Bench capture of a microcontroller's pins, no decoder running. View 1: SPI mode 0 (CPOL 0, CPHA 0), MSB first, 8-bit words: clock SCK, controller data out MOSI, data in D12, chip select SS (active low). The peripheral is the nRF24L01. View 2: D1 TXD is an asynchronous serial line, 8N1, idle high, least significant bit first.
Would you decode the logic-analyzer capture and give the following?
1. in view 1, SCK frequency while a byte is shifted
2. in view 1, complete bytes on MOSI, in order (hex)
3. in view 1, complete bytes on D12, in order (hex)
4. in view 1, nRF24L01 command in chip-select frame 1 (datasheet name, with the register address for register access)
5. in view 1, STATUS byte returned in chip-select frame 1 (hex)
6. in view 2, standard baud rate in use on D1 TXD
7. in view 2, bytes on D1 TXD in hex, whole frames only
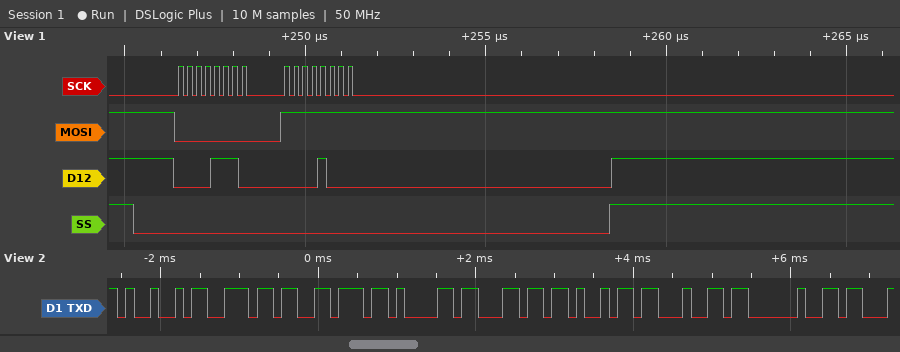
4 MHz
00 FF
0E 08
R_REGISTER 0x00
0x0E
9600 baud
0x49 0x6E 0x76 0x61 0x6C 0x69 0x64 0x20
